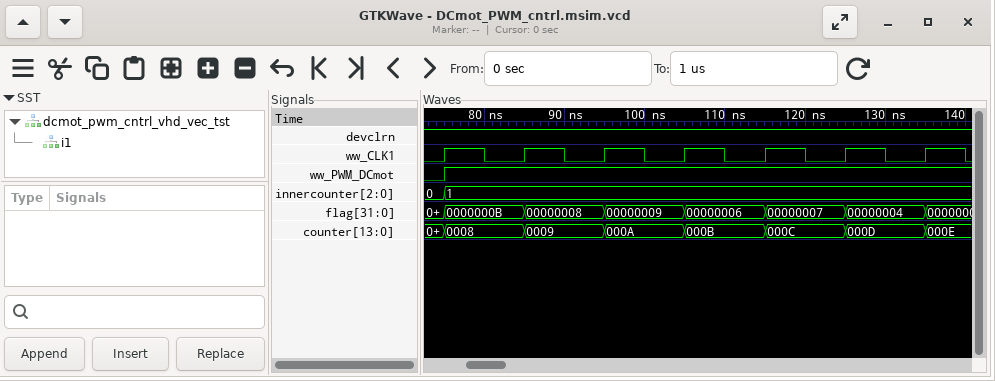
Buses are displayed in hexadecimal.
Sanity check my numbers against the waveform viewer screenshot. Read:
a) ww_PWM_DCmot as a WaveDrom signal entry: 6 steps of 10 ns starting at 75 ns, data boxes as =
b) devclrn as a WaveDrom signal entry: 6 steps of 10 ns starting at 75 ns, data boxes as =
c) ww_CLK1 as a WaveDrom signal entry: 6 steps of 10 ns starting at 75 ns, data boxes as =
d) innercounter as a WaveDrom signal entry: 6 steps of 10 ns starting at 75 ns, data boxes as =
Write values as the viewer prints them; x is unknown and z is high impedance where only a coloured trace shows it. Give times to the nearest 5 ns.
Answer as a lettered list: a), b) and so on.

a) {name: 'ww_PWM_DCmot', wave: '1.....'}
b) {name: 'devclrn', wave: '1.....'}
c) {name: 'ww_CLK1', wave: 'p.....'}
d) {name: 'innercounter', wave: '=.....', data: '1'}
